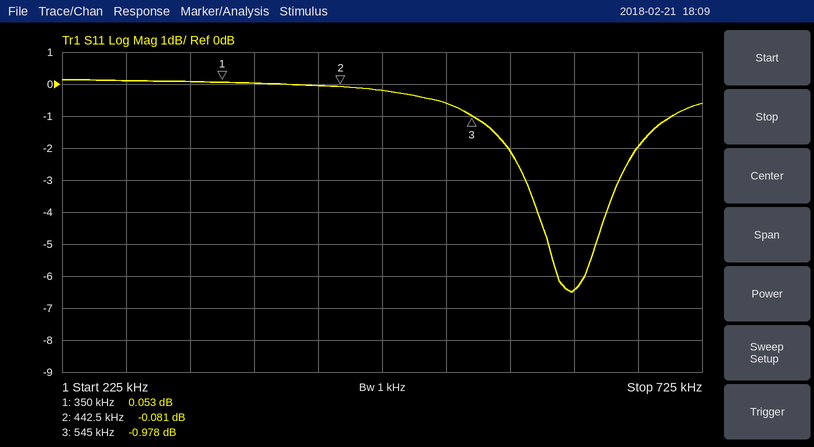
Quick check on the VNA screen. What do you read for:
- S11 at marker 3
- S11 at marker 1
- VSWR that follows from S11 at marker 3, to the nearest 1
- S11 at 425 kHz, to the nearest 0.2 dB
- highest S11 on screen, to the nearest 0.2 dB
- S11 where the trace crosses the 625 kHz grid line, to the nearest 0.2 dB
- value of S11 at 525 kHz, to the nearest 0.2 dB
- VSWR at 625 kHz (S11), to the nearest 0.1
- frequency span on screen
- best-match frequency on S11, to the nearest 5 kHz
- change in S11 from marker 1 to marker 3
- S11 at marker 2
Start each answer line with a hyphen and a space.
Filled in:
- -0.978 dB
- 0.053 dB
- 18
- 0.0 dB
- 0.2 dB
- -6.4 dB
- -0.6 dB
- 2.8
- 500 kHz
- 625 kHz
- -1.031 dB
- -0.081 dB
